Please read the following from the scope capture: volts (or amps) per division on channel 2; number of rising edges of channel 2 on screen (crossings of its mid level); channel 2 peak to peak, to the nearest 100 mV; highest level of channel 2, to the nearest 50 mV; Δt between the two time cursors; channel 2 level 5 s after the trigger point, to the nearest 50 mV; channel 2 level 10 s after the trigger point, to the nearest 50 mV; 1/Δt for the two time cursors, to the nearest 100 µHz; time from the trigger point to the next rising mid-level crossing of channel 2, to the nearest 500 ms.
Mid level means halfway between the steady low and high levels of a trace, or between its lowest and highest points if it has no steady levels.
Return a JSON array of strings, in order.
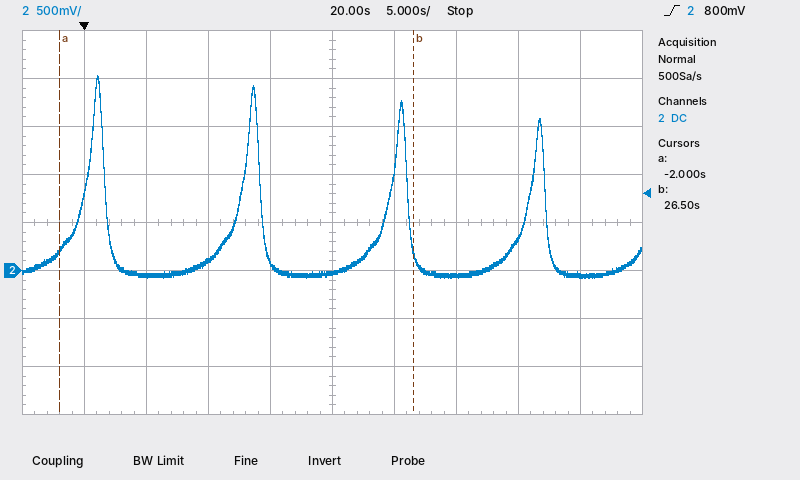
["500 mV", "4", "2.10 V", "2.05 V", "28.5 s", "-50 mV", "100 mV", "35.1 mHz", "500 ms"]
